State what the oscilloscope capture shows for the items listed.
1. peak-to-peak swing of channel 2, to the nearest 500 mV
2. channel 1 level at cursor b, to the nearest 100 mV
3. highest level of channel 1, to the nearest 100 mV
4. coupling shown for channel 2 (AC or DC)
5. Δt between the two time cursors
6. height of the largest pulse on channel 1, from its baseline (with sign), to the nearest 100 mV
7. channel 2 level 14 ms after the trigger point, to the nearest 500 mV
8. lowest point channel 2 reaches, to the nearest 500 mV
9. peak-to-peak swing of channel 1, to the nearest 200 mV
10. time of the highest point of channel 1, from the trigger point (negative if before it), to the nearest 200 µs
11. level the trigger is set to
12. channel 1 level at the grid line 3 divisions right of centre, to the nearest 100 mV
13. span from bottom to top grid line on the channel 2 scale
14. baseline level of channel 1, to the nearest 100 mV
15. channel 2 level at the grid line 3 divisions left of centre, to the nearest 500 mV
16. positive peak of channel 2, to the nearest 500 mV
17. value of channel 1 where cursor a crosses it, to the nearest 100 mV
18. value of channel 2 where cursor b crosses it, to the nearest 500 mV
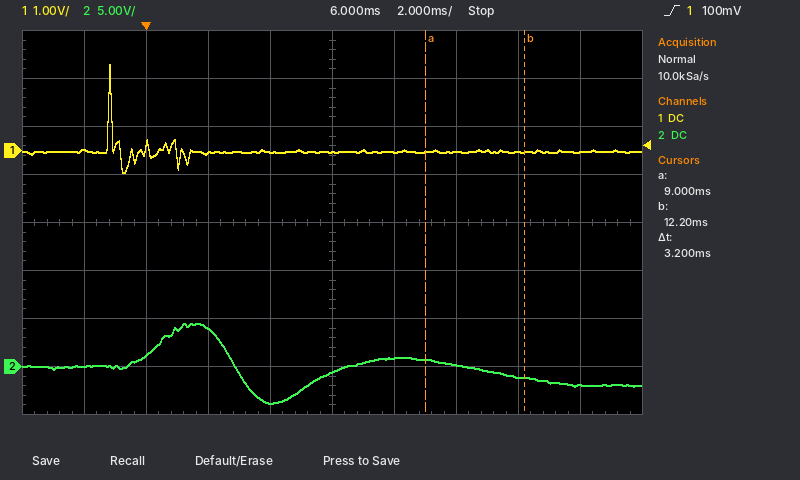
8.5 V
0.0 V
1.8 V
DC
3.2 ms
+1.8 V
-2.0 V
-4.0 V
2.2 V
-1.2 ms
100 mV
0.0 V
40 V
0.0 V
1.0 V
4.5 V
0.0 V
-1.0 V
